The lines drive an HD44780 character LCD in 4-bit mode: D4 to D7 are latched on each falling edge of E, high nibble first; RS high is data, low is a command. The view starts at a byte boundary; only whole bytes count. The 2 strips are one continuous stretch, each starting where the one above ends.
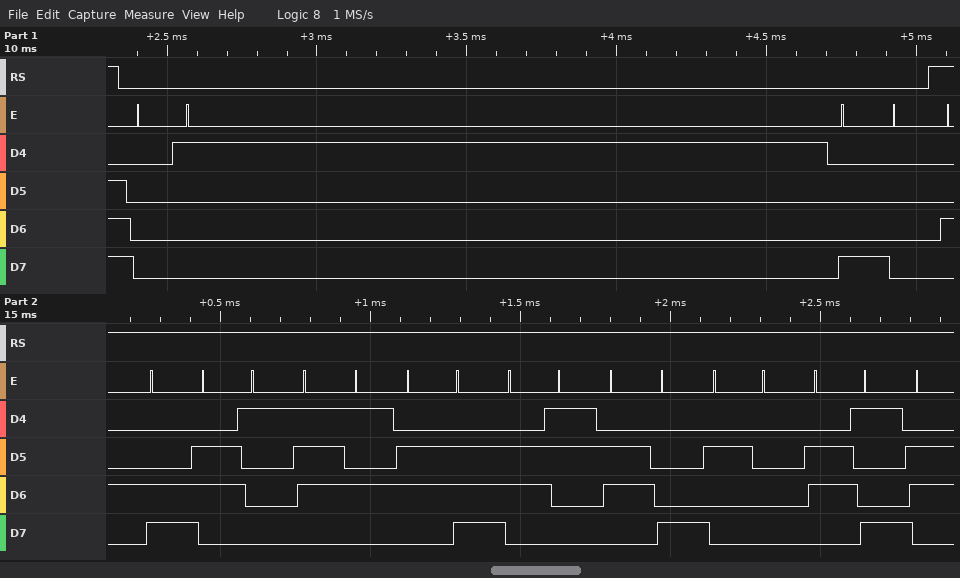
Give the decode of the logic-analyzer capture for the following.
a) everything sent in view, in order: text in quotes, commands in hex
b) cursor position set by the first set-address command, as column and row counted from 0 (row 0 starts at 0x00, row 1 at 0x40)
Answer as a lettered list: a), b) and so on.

a) 0x01 0x80 "Launch i"
b) column 0, row 0
